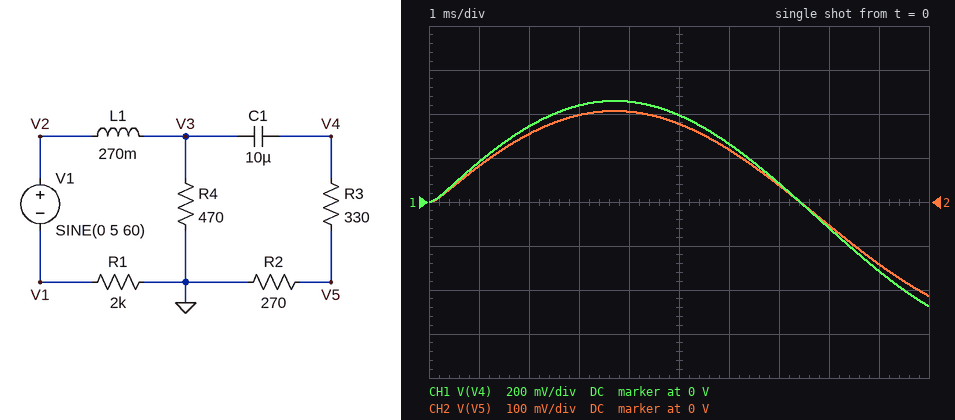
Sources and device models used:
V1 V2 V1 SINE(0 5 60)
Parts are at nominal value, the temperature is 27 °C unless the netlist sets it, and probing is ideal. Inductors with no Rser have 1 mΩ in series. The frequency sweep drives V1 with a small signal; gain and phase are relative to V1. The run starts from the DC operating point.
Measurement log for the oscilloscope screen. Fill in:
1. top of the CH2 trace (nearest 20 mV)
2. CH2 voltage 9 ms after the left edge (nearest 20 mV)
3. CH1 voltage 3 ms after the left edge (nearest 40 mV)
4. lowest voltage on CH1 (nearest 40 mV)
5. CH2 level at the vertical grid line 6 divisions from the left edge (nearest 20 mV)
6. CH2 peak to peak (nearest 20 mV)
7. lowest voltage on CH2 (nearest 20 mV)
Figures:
200 mV
-140 mV
440 mV
-480 mV
120 mV
420 mV
-220 mV
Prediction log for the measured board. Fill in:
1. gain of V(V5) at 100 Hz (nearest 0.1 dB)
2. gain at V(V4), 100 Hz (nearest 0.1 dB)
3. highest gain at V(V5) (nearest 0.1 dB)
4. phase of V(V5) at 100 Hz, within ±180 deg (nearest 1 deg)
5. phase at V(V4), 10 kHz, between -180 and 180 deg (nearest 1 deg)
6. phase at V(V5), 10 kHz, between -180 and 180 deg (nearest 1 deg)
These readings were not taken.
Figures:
-25.7 dB
-18.8 dB
-25.7 dB
5 deg
-82 deg
-82 deg
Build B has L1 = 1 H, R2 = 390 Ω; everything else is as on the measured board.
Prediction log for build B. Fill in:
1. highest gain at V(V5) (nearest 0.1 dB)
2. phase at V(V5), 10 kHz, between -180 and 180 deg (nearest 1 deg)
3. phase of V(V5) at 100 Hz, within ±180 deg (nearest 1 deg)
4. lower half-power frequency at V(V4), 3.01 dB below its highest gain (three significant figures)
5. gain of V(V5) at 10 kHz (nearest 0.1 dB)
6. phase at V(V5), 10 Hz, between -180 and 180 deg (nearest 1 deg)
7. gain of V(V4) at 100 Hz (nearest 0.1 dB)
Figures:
-23.7 dB
-88 deg
-7 deg
13.5 Hz
-52.2 dB
54 deg
-18.5 dB
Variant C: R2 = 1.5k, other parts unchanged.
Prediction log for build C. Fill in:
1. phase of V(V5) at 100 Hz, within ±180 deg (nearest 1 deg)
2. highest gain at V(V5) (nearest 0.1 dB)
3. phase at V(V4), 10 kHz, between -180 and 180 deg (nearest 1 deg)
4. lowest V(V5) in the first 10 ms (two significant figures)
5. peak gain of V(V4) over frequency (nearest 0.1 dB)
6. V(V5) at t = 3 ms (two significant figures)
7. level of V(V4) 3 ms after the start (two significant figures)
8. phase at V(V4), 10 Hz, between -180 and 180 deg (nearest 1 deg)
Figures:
0 deg
-17.8 dB
-82 deg
-460 mV
-16.1 dB
530 mV
650 mV
35 deg
